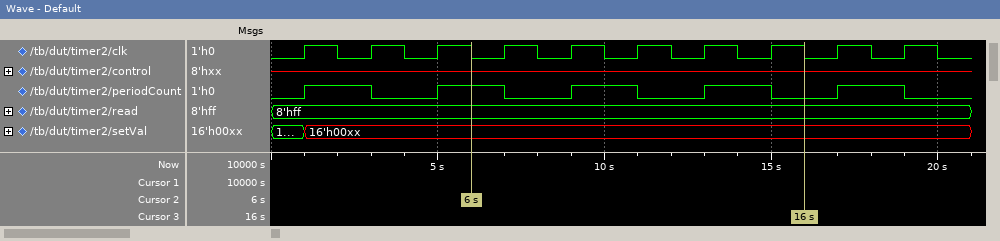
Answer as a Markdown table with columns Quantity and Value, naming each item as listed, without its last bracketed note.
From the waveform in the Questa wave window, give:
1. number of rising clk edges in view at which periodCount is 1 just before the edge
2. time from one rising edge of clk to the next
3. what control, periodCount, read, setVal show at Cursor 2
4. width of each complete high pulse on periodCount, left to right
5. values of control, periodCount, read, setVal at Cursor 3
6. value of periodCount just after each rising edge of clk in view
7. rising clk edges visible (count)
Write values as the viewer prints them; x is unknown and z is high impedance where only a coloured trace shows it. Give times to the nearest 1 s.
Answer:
| Quantity | Value |
|---|---|
| number of rising clk edges in view at which periodCount is 1 just before the edge | 5 |
| time from one rising edge of clk to the next | 2 s |
| what control, periodCount, read, setVal show at Cursor 2 | control=x, periodCount=1, read=8'hff, setVal=16'h00xx |
| width of each complete high pulse on periodCount, left to right | 2 s, 2 s, 2 s, 2 s, 2 s |
| values of control, periodCount, read, setVal at Cursor 3 | control=x, periodCount=0, read=8'hff, setVal=16'h00xx |
| value of periodCount just after each rising edge of clk in view | 1 0 1 0 1 0 1 0 1 0 |
| rising clk edges visible | 10 |
